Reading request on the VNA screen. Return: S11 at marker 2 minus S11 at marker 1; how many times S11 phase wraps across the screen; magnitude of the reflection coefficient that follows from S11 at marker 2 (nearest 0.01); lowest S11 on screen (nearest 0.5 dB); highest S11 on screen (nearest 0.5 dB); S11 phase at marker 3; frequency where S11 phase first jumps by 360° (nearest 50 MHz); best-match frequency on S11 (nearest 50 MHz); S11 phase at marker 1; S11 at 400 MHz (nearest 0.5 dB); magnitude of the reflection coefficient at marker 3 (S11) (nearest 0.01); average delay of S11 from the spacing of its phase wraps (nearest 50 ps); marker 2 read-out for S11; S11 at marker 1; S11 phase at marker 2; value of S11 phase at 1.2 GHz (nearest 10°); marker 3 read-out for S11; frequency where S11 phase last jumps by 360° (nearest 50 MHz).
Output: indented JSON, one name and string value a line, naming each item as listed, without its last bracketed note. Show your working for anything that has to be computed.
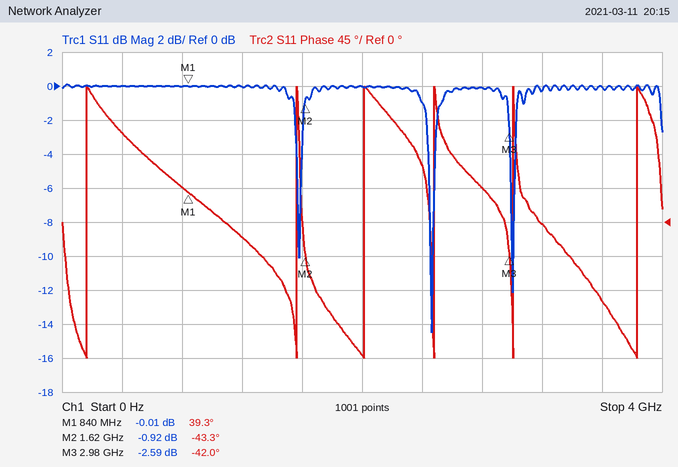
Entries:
{
  "S11 at marker 2 minus S11 at marker 1": "-0.92 − (-0.01) = -0.91 dB",
  "how many times S11 phase wraps across the screen": "6",
  "magnitude of the reflection coefficient that follows from S11 at marker 2": "10^(-0.92/20) ≈ 0.90",
  "lowest S11 on screen": "-14.5 dB",
  "highest S11 on screen": "0.0 dB",
  "S11 phase at marker 3": "-42.0°",
  "frequency where S11 phase first jumps by 360°": "150 MHz",
  "best-match frequency on S11": "2.45 GHz",
  "S11 phase at marker 1": "39.3°",
  "S11 at 400 MHz": "0.0 dB",
  "magnitude of the reflection coefficient at marker 3 (S11)": "10^(-2.59/20) ≈ 0.74",
  "average delay of S11 from the spacing of its phase wraps": "5 cycles / (3.85 GHz − 150 MHz) ≈ 1.35 ns",
  "marker 2 read-out for S11": "-0.92 dB",
  "S11 at marker 1": "-0.01 dB",
  "S11 phase at marker 2": "-43.3°",
  "value of S11 phase at 1.2 GHz": "-20°",
  "marker 3 read-out for S11": "-2.59 dB",
  "frequency where S11 phase last jumps by 360°": "3.85 GHz"
}
